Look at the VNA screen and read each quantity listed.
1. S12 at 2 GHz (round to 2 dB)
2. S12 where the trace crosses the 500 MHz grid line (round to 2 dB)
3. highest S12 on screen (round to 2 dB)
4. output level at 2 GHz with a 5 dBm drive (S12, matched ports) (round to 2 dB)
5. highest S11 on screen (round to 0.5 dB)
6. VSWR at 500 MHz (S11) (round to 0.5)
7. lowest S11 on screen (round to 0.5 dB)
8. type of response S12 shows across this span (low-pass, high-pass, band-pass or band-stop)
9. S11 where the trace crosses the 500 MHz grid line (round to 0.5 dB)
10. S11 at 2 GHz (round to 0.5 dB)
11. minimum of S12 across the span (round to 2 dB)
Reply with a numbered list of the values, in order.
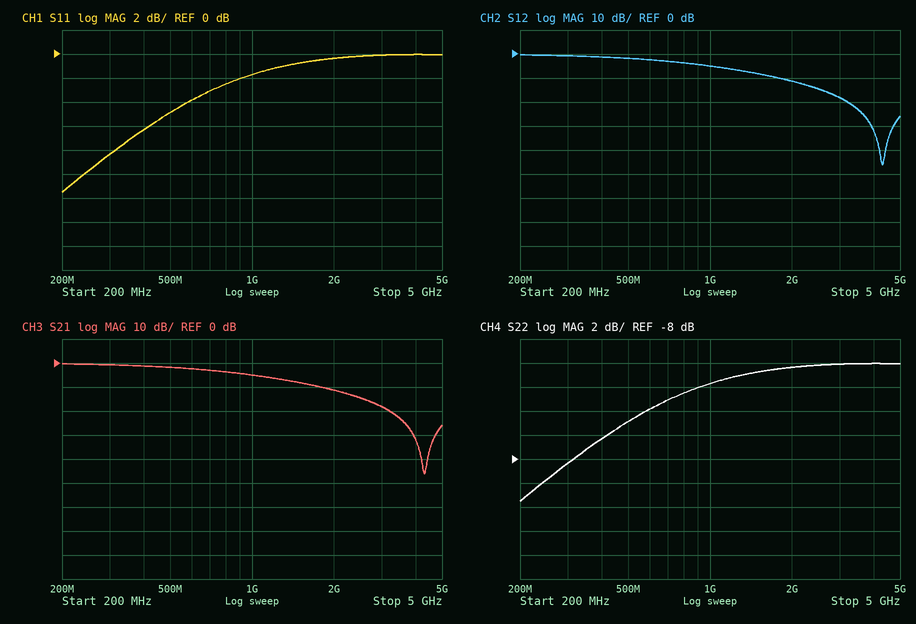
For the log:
1. -12 dB
2. -2 dB
3. 0 dB
4. -6 dBm
5. 0.0 dB
6. 3.5
7. -11.5 dB
8. low-pass
9. -5.0 dB
10. -0.5 dB
11. -46 dB
